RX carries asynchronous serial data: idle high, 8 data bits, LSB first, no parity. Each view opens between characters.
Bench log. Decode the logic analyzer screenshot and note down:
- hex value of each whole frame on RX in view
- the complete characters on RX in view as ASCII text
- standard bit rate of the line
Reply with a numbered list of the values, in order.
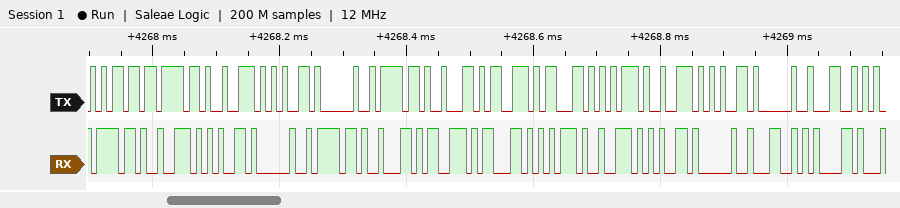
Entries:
1. 6F, 72, 65, 20, 6F, 62, 73, 63, 75, 72, 65, 20, 4C, 61
2. "ore obscure La"
3. 115200 baud
